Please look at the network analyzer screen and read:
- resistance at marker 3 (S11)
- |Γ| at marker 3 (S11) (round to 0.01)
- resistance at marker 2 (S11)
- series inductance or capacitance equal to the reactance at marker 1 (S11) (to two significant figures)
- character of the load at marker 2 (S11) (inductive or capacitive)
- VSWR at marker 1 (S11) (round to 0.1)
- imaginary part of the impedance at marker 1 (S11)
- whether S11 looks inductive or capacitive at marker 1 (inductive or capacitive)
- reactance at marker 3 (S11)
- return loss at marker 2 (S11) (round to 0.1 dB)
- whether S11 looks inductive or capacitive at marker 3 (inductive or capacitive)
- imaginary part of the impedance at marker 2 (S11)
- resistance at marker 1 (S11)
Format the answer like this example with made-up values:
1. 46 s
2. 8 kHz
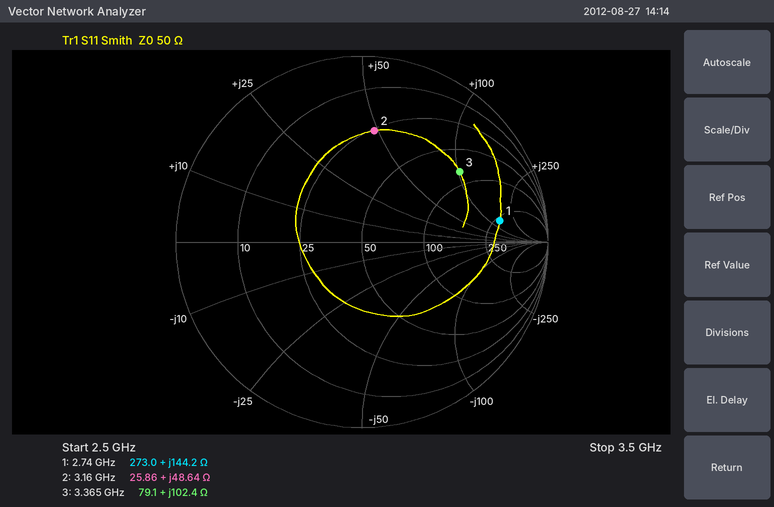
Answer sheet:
1. 79.1 Ω
2. 0.65
3. 25.86 Ω
4. 8.4 nH
5. inductive
6. 7.0
7. +144.2 Ω
8. inductive
9. +102.4 Ω
10. 4.4 dB
11. inductive
12. +48.64 Ω
13. 273.0 Ω
